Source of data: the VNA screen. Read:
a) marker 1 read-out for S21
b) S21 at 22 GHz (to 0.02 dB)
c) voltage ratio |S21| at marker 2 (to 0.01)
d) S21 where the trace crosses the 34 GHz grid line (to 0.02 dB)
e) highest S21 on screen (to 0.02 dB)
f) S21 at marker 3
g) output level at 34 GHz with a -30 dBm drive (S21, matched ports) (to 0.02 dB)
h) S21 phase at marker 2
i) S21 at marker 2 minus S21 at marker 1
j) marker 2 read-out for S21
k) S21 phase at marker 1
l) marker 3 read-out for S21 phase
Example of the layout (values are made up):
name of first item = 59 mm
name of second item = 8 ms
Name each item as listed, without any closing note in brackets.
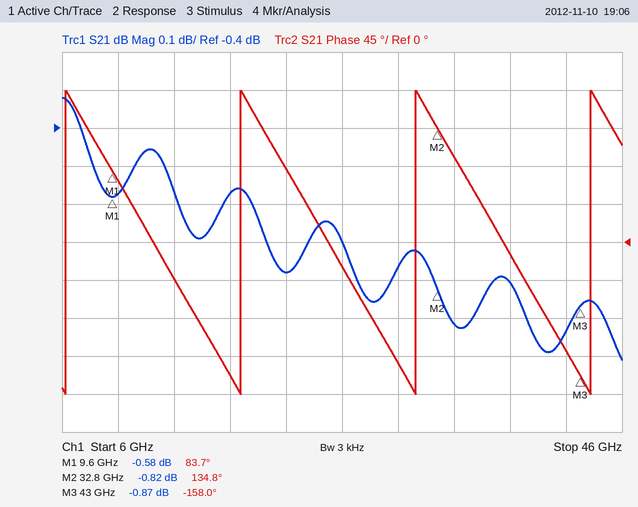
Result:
marker 1 read-out for S21 = -0.58 dB
S21 at 22 GHz = -0.78 dB
voltage ratio |S21| at marker 2 = 0.91
S21 where the trace crosses the 34 GHz grid line = -0.92 dB
highest S21 on screen = -0.32 dB
S21 at marker 3 = -0.87 dB
output level at 34 GHz with a -30 dBm drive (S21, matched ports) = -30.92 dBm
S21 phase at marker 2 = 134.8°
S21 at marker 2 minus S21 at marker 1 = -0.24 dB
marker 2 read-out for S21 = -0.82 dB
S21 phase at marker 1 = 83.7°
marker 3 read-out for S21 phase = -158.0°
